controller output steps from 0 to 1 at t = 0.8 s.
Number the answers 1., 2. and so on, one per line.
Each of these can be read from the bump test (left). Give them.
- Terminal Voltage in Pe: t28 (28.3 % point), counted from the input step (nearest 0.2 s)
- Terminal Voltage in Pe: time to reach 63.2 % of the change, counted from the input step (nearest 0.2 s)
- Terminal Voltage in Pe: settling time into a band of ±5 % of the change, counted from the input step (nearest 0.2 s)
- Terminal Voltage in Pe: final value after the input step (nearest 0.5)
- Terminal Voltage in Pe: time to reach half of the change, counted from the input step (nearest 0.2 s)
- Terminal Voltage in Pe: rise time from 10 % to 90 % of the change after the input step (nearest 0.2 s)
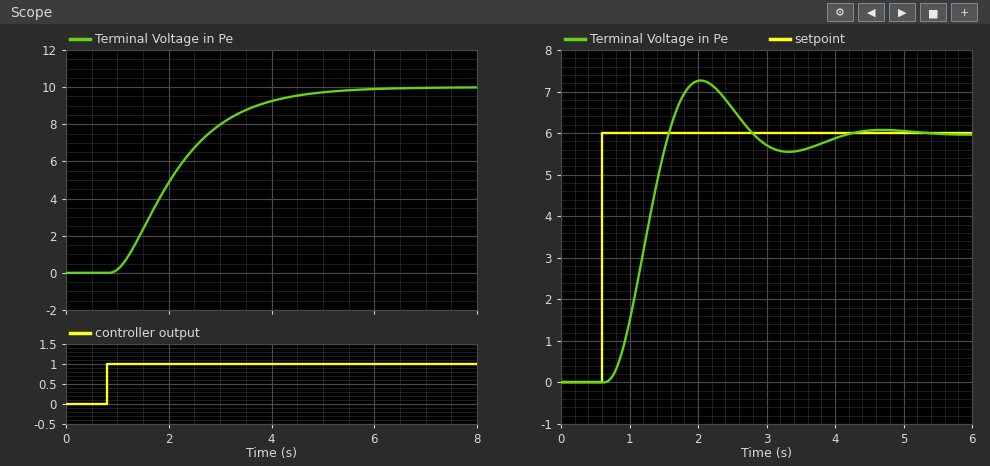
1. 0.8 s
2. 1.6 s
3. 3.6 s
4. 10.0
5. 1.2 s
6. 2.4 s
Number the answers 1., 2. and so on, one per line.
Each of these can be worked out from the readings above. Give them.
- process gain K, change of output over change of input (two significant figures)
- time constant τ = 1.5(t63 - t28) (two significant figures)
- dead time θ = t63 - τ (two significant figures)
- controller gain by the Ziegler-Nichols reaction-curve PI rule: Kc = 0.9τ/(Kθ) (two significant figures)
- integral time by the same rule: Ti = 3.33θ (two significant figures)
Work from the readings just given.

1. 10
2. 1.2 s
3. 0.40 s
4. 0.27
5. 1.3 s
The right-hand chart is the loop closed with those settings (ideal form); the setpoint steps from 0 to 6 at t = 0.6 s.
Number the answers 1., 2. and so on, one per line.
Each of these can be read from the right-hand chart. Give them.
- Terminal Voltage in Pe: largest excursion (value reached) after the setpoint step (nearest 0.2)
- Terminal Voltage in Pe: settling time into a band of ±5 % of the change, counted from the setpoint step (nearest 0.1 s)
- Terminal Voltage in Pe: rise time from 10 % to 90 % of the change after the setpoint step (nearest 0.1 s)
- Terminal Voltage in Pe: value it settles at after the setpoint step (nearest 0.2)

1. 7.2
2. 3.1 s
3. 0.6 s
4. 6.0
